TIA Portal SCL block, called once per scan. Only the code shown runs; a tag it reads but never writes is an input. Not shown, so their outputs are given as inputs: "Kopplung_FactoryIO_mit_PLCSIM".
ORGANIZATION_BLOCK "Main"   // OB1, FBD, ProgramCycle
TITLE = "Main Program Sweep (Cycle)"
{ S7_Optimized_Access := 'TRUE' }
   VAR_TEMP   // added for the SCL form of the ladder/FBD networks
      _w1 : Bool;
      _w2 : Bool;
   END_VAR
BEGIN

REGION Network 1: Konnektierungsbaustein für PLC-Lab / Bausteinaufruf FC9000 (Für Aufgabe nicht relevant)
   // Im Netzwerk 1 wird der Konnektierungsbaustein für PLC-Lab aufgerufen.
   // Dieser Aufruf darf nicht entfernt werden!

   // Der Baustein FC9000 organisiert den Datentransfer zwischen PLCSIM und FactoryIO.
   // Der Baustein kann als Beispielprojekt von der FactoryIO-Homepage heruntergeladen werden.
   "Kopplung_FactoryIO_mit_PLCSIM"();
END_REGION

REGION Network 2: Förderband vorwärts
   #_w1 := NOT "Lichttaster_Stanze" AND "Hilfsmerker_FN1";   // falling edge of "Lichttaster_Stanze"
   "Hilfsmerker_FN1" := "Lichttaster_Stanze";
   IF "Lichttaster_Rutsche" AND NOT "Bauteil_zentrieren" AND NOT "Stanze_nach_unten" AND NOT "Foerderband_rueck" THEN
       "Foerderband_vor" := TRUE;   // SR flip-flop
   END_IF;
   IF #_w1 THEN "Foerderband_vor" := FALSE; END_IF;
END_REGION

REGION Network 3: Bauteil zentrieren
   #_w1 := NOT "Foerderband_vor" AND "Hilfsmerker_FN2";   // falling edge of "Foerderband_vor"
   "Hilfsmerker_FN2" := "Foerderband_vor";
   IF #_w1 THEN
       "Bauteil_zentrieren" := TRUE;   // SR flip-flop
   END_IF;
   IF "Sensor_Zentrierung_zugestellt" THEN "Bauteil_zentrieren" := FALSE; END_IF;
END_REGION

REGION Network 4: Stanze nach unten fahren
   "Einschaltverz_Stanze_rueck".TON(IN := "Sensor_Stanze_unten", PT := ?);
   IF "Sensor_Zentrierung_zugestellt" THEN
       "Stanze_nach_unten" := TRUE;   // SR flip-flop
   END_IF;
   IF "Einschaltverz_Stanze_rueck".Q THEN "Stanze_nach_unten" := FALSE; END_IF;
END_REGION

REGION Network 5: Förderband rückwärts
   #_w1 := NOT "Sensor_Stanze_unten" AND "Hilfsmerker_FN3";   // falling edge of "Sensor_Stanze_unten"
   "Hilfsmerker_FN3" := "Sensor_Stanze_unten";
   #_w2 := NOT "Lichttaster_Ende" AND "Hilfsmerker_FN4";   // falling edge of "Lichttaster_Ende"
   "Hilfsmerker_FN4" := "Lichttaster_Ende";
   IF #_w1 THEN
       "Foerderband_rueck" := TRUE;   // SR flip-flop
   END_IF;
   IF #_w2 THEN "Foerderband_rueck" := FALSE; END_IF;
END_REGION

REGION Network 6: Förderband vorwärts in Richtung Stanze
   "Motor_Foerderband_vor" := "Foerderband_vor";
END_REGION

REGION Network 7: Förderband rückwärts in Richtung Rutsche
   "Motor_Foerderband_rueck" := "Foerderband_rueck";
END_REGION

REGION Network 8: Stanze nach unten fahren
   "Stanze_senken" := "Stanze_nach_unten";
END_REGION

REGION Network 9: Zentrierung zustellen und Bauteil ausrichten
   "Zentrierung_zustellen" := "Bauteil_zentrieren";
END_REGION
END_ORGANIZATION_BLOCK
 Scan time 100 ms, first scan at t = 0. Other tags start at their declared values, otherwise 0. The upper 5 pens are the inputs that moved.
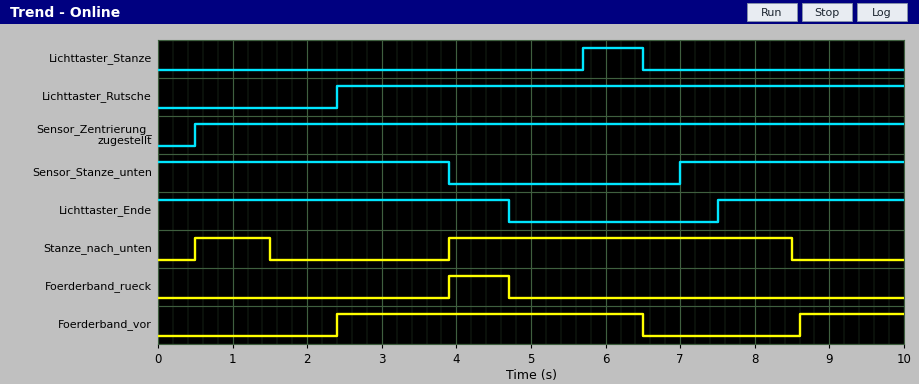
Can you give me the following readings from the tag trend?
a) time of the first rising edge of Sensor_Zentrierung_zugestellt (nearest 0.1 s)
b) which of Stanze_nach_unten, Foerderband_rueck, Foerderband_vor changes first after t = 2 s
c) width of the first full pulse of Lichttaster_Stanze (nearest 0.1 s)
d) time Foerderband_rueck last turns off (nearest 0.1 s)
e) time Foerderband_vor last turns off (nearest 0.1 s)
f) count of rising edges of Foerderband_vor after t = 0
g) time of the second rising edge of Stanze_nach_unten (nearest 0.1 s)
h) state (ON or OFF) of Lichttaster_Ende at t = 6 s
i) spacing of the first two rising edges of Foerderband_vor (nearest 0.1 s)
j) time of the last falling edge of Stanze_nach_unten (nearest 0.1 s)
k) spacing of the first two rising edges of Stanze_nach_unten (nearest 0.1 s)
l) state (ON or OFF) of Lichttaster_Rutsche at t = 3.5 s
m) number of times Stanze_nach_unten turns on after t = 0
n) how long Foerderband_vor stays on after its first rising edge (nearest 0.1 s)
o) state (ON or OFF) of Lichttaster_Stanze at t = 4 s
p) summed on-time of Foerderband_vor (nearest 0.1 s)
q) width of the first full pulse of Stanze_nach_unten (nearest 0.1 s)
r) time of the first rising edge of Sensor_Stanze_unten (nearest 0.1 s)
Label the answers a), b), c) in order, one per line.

a) 0.5 s
b) Foerderband_vor
c) 0.8 s
d) 4.7 s
e) 6.5 s
f) 2
g) 3.9 s
h) OFF
i) 6.2 s
j) 8.5 s
k) 3.4 s
l) ON
m) 2
n) 4.1 s
o) OFF
p) 5.5 s
q) 1.0 s
r) 7.0 s
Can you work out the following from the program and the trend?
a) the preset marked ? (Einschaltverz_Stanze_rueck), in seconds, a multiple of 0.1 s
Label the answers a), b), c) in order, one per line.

a) 1.5 s
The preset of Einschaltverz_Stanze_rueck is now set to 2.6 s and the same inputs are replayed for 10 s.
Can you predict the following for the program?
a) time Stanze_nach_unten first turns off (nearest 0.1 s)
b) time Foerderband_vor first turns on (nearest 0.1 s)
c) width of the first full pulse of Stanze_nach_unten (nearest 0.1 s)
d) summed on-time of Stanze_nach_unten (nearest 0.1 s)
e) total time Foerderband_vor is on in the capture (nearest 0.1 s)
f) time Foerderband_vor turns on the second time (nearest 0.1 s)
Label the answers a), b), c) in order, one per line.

a) 2.6 s
b) 2.7 s
c) 2.1 s
d) 7.8 s
e) 4.1 s
f) 9.7 s
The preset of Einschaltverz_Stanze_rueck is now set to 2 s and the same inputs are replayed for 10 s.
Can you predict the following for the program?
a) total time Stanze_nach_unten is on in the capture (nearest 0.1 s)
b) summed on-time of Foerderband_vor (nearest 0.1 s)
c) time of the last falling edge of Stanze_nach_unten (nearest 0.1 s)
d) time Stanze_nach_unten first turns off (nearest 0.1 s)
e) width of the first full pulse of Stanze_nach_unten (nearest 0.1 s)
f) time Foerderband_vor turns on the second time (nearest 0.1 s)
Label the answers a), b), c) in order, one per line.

a) 6.6 s
b) 5.0 s
c) 9.0 s
d) 2.0 s
e) 1.5 s
f) 9.1 s
